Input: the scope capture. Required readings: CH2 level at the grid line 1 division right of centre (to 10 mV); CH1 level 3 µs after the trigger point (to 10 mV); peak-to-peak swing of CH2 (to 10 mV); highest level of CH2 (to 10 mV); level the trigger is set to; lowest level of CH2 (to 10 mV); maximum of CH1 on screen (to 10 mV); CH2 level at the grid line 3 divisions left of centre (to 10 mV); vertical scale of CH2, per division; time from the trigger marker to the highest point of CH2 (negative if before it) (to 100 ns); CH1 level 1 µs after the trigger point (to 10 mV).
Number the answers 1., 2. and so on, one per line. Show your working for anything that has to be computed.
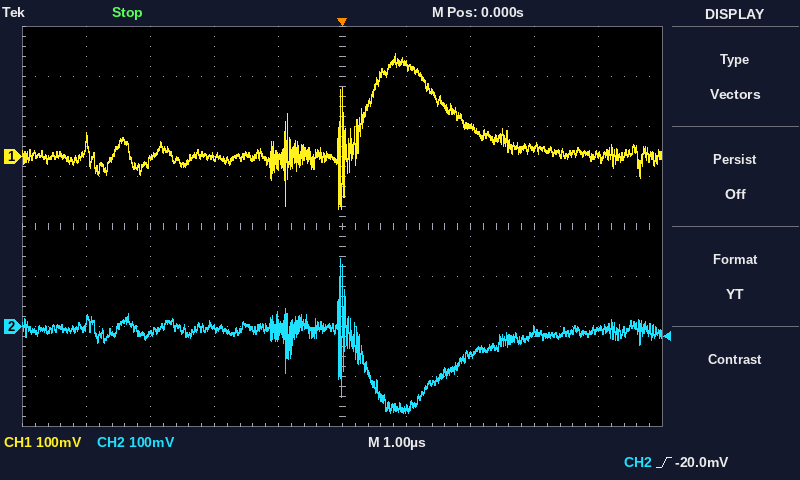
1. -160 mV
2. 20 mV
3. 140 mV − (-170 mV) = 310 mV
4. 140 mV
5. -20.0 mV
6. -170 mV
7. 210 mV
8. -10 mV
9. 100 mV
10. 0.0 µs
11. 180 mV
